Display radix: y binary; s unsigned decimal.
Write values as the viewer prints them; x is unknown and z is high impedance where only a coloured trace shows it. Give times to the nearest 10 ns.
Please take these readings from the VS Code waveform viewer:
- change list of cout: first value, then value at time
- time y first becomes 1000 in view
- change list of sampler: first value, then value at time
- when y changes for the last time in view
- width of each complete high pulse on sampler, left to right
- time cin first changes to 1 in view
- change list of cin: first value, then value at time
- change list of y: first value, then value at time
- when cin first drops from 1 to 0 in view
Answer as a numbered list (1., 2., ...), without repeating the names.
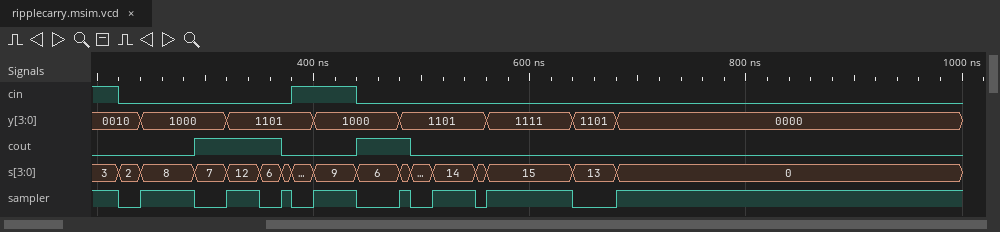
1. 0, 1 at 290 ns, 0 at 370 ns, 1 at 440 ns, 0 at 490 ns
2. 240 ns
3. 1, 0 at 220 ns, 1 at 240 ns, 0 at 290 ns, 1 at 320 ns, 0 at 350 ns, 1 at 370 ns, 0 at 380 ns, 1 at 400 ns, 0 at 440 ns, 1 at 480 ns, 0 at 490 ns, 1 at 510 ns, 0 at 550 ns, 1 at 560 ns, 0 at 640 ns, 1 at 680 ns
4. 680 ns
5. 50 ns, 30 ns, 10 ns, 40 ns, 10 ns, 40 ns, 80 ns
6. 380 ns
7. 1, 0 at 220 ns, 1 at 380 ns, 0 at 440 ns
8. 0010, 1000 at 240 ns, 1101 at 320 ns, 1000 at 400 ns, 1101 at 480 ns, 1111 at 560 ns, 1101 at 640 ns, 0000 at 680 ns
9. 220 ns
